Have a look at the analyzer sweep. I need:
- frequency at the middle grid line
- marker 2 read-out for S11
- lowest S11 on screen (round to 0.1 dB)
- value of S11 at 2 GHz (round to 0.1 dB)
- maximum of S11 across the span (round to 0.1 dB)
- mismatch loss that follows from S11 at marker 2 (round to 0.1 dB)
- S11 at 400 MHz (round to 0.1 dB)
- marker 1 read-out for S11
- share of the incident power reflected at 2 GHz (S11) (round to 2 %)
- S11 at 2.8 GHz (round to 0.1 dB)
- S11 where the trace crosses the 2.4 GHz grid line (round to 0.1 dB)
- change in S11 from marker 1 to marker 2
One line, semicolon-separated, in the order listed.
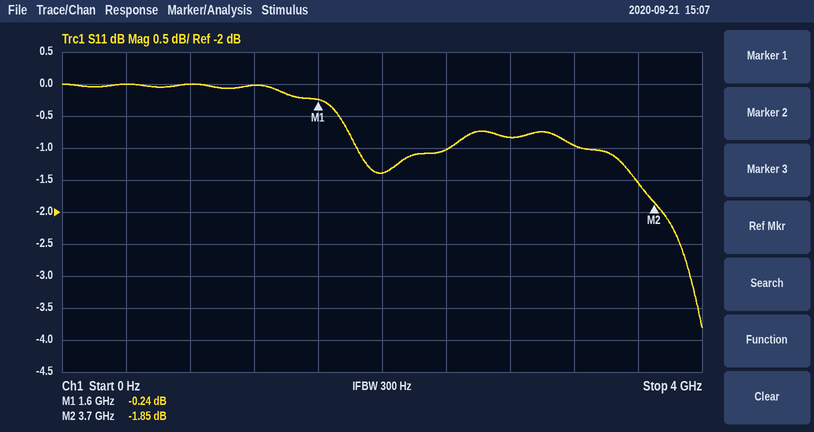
2 GHz; -1.85 dB; -3.8 dB; -1.4 dB; 0.0 dB; 4.6 dB; 0.0 dB; -0.24 dB; 72 %; -0.8 dB; -1.0 dB; -1.61 dB
